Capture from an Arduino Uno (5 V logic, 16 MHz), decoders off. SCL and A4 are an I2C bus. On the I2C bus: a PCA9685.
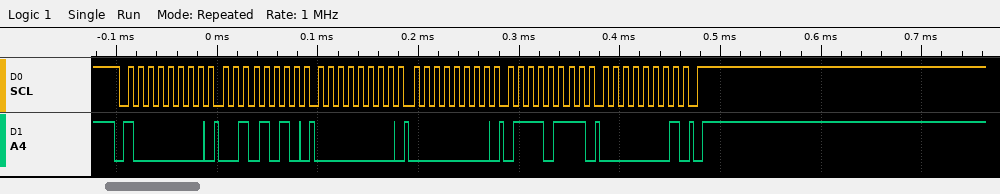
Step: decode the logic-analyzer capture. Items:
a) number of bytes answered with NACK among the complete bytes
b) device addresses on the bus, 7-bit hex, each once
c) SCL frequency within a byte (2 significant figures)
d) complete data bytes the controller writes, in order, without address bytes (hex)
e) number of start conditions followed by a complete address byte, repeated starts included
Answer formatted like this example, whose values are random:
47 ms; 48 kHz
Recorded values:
0; 0x40; 100 kHz; 2A 00 00 77 01; 1
